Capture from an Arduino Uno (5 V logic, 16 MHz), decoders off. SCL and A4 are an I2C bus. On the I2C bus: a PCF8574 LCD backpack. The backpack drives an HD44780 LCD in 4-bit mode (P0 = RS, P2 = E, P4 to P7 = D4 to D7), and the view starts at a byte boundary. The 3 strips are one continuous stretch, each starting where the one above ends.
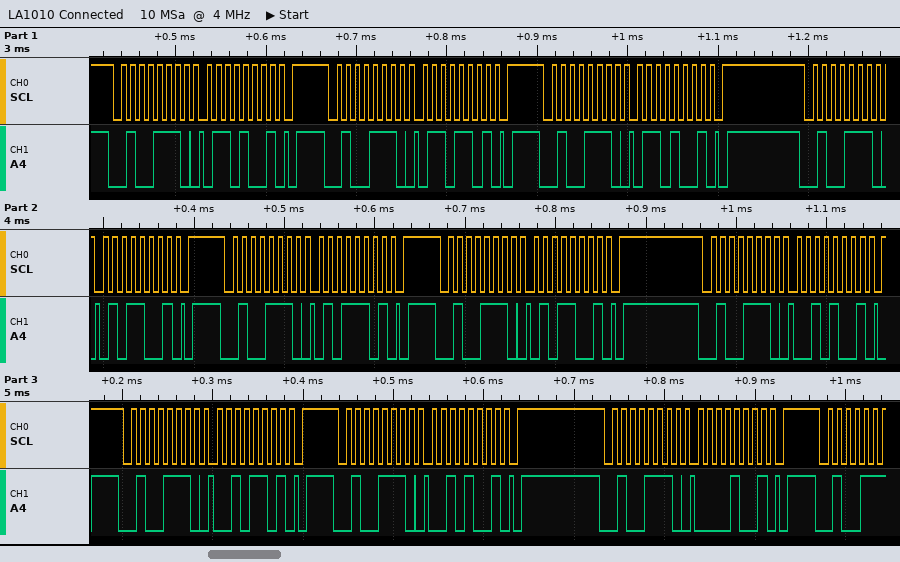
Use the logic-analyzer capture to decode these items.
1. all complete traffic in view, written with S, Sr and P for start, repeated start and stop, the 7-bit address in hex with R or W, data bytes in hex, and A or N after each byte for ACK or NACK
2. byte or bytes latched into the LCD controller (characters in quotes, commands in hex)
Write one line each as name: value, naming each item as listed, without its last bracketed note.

all complete traffic in view, written with S, Sr and P for start, repeated start and stop, the 7-bit address in hex with R or W, data bytes in hex, and A or N after each byte for ACK or NACK: S 27W A 69 A P S 27W A 6D A P S 27W A 69 A P S 27W A 59 A P S 27W A 5D A P S 27W A 59 A P S 27W A 29 A P S 27W A 2D A P S 27W A 29 A P S 27W A 09 A P
byte or bytes latched into the LCD controller: 'e'
